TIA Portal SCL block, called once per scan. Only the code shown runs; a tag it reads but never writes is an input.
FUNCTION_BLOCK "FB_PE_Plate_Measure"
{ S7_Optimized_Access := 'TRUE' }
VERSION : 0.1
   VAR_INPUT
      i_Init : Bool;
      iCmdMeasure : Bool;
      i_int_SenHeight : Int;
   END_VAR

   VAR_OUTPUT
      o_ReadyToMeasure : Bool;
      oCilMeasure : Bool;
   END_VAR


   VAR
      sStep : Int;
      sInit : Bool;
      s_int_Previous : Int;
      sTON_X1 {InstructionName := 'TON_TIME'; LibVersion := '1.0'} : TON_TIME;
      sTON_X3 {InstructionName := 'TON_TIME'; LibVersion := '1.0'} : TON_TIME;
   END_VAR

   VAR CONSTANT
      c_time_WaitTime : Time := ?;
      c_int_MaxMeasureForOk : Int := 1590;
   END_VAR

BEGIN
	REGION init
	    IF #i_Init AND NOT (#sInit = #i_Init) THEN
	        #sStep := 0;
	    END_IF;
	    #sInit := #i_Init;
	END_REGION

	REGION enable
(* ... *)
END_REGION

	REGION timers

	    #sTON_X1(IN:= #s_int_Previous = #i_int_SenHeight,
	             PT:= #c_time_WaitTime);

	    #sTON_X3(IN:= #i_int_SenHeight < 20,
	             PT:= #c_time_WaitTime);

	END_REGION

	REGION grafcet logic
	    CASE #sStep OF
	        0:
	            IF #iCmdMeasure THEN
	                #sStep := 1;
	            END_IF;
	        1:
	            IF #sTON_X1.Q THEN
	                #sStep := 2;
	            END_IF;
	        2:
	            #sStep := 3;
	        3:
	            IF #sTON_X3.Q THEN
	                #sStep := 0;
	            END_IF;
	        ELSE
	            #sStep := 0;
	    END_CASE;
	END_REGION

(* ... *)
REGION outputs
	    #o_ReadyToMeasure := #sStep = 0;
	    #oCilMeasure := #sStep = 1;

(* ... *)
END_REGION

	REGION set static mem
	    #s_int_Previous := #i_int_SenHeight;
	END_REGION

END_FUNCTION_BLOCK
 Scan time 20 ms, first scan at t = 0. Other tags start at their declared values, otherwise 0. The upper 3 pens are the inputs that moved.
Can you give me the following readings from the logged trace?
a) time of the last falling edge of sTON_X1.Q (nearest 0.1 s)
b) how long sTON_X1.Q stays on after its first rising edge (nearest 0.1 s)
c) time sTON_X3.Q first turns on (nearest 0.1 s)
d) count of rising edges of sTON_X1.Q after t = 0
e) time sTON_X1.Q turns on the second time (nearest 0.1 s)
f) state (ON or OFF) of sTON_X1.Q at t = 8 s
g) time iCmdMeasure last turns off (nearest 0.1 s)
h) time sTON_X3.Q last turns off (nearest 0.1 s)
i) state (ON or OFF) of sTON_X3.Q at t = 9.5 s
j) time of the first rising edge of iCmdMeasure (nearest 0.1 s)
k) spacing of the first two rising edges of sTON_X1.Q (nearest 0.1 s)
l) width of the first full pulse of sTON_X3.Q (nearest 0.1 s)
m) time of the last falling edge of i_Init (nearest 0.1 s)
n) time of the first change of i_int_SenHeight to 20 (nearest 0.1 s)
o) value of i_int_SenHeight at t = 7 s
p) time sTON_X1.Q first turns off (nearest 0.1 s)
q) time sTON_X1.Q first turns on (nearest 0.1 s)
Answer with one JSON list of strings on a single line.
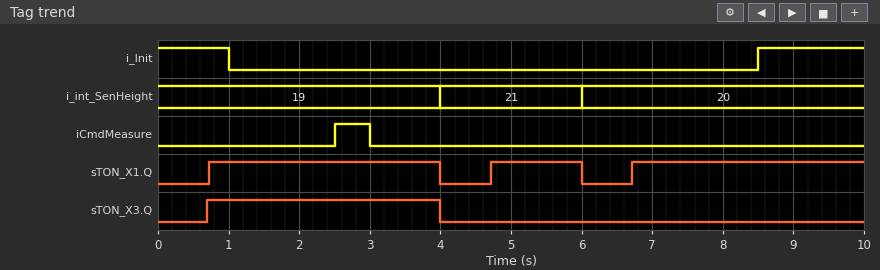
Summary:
["6.0 s", "3.3 s", "0.7 s", "3", "4.7 s", "ON", "3.0 s", "4.0 s", "OFF", "2.5 s", "4.0 s", "3.3 s", "1.0 s", "6.0 s", "20", "4.0 s", "0.7 s"]
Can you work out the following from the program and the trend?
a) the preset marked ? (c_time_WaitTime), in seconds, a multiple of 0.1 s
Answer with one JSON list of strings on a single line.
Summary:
["0.7 s"]
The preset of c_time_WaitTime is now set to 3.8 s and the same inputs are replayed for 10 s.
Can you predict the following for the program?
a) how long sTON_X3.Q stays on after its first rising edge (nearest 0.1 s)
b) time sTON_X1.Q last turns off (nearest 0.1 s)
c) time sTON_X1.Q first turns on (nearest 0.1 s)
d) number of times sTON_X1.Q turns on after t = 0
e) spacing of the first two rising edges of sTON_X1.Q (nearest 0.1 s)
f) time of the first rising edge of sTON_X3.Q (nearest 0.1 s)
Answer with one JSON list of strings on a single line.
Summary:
["0.2 s", "4.0 s", "3.8 s", "2", "6.0 s", "3.8 s"]
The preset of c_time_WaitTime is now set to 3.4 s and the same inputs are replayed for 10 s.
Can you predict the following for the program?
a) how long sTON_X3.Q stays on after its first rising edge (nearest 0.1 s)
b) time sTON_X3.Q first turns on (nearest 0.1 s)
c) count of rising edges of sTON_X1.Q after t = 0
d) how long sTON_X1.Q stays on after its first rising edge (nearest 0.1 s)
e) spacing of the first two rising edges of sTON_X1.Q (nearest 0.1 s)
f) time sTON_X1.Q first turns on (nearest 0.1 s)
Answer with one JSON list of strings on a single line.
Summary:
["0.6 s", "3.4 s", "2", "0.6 s", "6.0 s", "3.4 s"]
